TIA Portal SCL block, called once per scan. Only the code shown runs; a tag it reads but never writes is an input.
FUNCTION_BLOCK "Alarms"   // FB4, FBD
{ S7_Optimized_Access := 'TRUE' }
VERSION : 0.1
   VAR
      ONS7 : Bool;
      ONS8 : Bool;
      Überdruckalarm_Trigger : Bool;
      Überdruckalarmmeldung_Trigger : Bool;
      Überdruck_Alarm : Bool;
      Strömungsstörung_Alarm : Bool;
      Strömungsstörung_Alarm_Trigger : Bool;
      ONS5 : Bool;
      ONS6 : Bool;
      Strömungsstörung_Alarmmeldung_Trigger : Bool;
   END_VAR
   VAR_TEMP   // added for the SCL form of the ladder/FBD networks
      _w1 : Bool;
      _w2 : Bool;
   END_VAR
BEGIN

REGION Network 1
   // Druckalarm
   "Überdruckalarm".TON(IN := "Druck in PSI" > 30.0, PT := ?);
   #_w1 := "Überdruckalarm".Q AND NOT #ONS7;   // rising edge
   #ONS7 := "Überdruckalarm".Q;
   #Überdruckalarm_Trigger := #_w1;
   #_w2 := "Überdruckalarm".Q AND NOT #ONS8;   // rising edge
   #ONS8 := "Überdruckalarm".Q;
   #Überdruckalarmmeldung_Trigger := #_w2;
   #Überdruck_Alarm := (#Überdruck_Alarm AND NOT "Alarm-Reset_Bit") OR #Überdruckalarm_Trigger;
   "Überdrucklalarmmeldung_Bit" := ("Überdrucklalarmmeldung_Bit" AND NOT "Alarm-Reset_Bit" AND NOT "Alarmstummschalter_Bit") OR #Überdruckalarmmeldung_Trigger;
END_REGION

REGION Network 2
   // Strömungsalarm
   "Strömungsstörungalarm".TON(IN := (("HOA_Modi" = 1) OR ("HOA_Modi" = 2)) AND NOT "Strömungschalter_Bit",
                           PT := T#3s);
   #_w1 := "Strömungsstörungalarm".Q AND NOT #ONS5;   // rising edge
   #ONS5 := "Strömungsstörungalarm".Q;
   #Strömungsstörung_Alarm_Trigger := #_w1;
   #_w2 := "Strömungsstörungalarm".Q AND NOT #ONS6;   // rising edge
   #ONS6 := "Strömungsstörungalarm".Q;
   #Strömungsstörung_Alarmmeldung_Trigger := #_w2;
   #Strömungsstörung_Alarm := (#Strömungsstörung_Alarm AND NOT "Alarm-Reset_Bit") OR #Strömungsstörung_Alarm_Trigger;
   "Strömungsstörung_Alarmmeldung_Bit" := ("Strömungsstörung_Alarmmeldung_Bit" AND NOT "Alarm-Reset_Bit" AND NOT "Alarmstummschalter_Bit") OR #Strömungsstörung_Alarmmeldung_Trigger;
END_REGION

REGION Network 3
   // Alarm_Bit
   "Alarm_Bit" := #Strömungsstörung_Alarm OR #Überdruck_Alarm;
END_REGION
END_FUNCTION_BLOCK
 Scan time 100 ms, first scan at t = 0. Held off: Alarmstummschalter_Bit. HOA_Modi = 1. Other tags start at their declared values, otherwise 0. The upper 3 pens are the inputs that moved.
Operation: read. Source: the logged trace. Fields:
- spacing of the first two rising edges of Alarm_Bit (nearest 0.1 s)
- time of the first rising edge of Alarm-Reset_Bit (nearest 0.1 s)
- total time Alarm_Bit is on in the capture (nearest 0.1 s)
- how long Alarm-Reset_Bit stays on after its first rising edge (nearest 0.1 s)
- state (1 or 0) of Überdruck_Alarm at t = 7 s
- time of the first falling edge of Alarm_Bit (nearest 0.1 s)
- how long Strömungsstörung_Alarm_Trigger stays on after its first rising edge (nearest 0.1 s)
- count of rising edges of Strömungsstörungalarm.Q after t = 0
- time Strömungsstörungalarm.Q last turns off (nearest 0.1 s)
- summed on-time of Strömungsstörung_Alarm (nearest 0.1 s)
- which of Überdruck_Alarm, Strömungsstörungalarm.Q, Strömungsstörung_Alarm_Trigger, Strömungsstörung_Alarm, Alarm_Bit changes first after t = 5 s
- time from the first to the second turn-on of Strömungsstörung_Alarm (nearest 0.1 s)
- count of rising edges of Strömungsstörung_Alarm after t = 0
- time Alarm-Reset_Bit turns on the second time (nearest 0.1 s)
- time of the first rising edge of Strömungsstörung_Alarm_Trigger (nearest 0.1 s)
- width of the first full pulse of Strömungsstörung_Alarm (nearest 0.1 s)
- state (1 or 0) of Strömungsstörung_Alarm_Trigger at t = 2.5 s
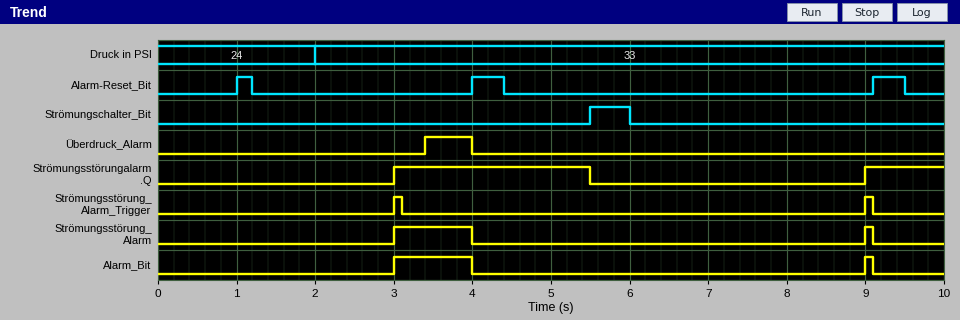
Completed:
6.0 s
1.0 s
1.1 s
0.2 s
0
4.0 s
0.1 s
2
5.5 s
1.1 s
Strömungsstörungalarm.Q
6.0 s
2
4.0 s
3.0 s
1.0 s
0
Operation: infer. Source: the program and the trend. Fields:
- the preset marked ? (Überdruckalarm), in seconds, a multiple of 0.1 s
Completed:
1.4 s
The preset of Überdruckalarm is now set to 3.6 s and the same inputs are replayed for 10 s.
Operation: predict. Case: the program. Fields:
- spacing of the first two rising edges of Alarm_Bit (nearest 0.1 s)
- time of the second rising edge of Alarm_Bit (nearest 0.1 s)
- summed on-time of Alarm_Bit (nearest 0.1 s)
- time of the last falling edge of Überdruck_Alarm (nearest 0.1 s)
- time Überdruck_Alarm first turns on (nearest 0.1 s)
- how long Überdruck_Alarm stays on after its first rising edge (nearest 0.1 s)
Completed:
2.6 s
5.6 s
4.5 s
9.1 s
5.6 s
3.5 s
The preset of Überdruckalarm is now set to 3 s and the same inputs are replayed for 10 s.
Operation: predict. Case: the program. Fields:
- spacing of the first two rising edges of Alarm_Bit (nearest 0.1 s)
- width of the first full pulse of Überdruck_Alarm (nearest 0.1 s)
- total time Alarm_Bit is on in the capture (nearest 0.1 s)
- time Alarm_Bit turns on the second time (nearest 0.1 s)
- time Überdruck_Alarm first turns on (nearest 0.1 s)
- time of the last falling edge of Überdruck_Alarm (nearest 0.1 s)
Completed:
2.0 s
4.1 s
5.1 s
5.0 s
5.0 s
9.1 s
